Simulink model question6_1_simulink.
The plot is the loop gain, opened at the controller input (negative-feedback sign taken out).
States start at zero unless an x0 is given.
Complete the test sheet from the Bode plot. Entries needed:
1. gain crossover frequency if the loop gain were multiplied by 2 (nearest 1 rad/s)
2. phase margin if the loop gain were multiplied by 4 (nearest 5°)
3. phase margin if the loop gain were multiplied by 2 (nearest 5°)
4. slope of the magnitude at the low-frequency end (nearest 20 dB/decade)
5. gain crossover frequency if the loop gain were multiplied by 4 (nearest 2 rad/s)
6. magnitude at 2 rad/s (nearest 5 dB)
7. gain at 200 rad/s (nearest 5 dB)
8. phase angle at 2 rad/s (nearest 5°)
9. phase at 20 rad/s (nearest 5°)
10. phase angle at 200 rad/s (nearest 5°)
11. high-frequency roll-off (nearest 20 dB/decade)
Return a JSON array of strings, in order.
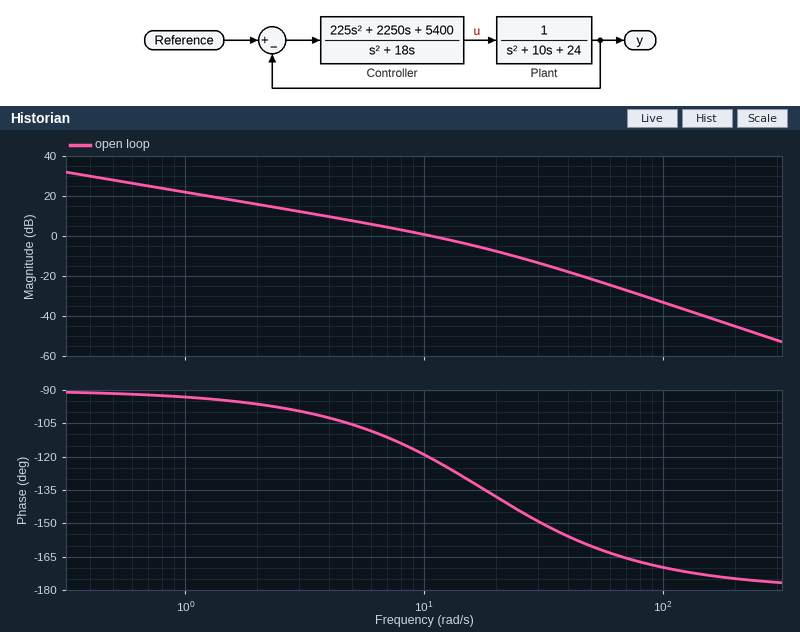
["18 rad/s", "35°", "45°", "-20 dB/decade", "28 rad/s", "15 dB", "-45 dB", "-95°", "-140°", "-175°", "-40 dB/decade"]
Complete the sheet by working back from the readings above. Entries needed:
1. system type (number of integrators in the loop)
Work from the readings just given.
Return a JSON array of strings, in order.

["1"]
